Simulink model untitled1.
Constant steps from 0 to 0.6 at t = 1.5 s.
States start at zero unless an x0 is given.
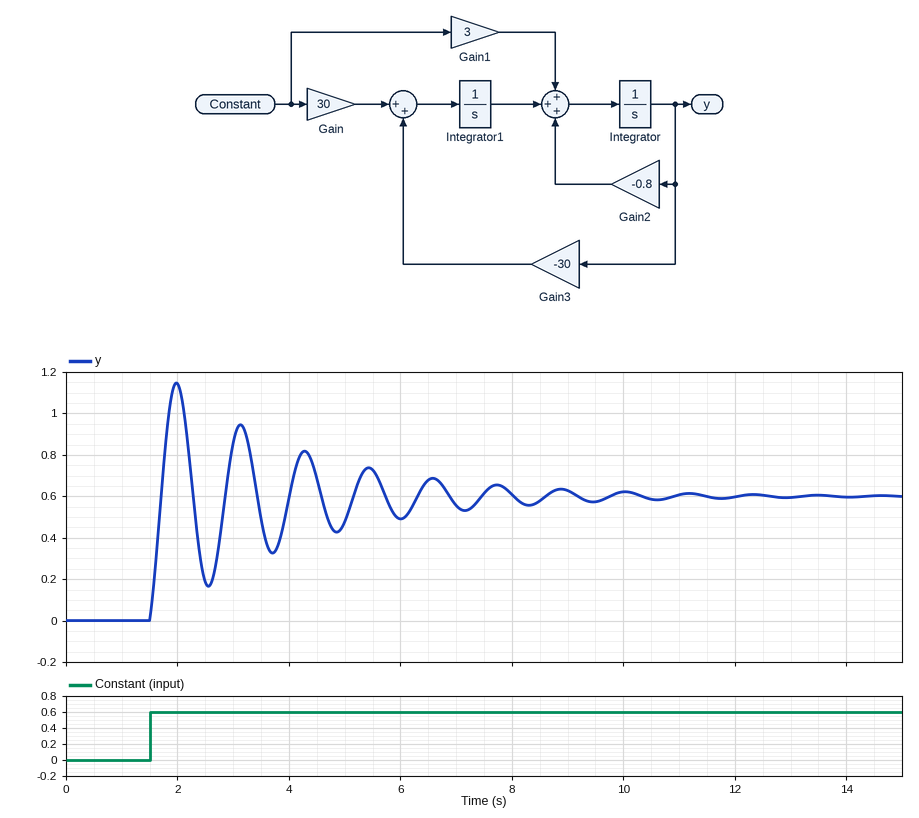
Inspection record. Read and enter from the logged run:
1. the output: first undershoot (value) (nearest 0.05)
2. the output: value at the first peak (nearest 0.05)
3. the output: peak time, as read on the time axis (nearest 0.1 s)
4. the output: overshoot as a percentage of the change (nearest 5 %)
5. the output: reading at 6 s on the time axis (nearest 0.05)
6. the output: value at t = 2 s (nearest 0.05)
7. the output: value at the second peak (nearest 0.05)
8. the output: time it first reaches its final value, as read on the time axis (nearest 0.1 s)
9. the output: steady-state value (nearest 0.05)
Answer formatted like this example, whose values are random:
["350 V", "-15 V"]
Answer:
["0.15", "1.15", "2.0 s", "90 %", "0.50", "1.15", "0.95", "1.7 s", "0.60"]
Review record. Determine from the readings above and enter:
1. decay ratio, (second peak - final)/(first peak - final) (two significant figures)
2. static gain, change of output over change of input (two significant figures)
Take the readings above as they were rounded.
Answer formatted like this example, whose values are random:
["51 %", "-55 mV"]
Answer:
["0.64", "1.0"]
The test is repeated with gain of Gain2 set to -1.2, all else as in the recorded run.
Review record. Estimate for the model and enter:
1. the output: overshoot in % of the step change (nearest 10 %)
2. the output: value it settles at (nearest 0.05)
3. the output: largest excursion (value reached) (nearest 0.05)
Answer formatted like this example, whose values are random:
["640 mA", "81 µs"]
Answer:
["80 %", "0.60", "1.10"]
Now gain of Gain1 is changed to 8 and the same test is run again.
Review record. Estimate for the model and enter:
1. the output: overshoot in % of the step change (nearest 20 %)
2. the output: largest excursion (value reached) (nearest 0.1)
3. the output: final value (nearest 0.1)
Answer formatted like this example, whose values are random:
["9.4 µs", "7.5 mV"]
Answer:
["140 %", "1.5", "0.6"]
